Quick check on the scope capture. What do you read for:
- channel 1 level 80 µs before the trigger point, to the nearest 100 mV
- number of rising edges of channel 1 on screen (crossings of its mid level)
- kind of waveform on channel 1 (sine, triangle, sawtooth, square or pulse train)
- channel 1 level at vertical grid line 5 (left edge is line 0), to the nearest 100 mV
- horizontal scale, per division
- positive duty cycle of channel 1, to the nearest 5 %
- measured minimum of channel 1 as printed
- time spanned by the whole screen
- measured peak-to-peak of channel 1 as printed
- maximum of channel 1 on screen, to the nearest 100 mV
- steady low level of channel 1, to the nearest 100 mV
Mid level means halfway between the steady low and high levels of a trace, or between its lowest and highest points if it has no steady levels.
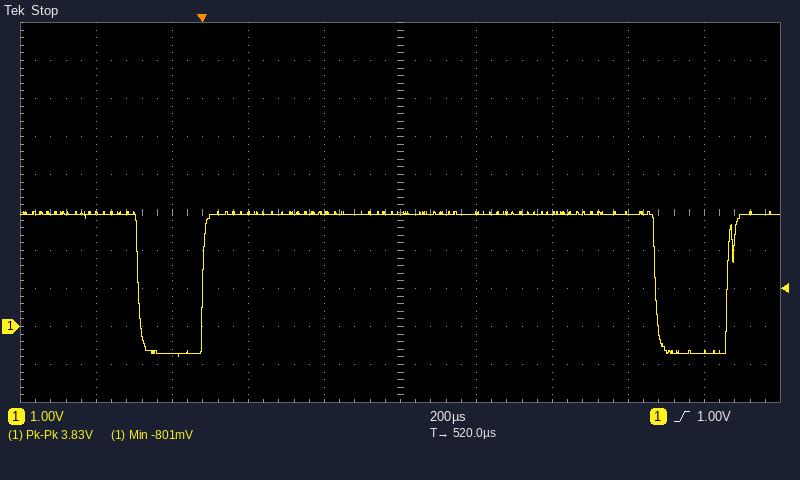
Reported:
-700 mV
2
pulse train
3.0 V
200 µs
85 %
-801 mV
2 ms
3.83 V
3.0 V
-700 mV
